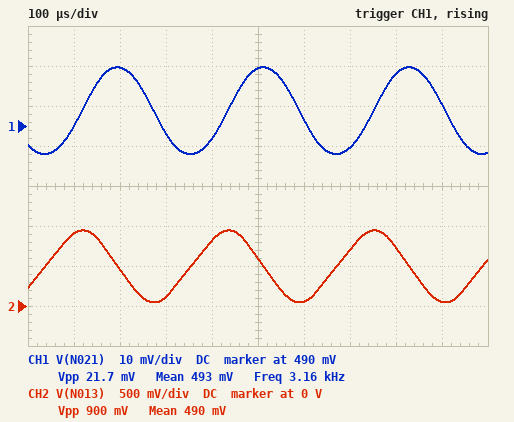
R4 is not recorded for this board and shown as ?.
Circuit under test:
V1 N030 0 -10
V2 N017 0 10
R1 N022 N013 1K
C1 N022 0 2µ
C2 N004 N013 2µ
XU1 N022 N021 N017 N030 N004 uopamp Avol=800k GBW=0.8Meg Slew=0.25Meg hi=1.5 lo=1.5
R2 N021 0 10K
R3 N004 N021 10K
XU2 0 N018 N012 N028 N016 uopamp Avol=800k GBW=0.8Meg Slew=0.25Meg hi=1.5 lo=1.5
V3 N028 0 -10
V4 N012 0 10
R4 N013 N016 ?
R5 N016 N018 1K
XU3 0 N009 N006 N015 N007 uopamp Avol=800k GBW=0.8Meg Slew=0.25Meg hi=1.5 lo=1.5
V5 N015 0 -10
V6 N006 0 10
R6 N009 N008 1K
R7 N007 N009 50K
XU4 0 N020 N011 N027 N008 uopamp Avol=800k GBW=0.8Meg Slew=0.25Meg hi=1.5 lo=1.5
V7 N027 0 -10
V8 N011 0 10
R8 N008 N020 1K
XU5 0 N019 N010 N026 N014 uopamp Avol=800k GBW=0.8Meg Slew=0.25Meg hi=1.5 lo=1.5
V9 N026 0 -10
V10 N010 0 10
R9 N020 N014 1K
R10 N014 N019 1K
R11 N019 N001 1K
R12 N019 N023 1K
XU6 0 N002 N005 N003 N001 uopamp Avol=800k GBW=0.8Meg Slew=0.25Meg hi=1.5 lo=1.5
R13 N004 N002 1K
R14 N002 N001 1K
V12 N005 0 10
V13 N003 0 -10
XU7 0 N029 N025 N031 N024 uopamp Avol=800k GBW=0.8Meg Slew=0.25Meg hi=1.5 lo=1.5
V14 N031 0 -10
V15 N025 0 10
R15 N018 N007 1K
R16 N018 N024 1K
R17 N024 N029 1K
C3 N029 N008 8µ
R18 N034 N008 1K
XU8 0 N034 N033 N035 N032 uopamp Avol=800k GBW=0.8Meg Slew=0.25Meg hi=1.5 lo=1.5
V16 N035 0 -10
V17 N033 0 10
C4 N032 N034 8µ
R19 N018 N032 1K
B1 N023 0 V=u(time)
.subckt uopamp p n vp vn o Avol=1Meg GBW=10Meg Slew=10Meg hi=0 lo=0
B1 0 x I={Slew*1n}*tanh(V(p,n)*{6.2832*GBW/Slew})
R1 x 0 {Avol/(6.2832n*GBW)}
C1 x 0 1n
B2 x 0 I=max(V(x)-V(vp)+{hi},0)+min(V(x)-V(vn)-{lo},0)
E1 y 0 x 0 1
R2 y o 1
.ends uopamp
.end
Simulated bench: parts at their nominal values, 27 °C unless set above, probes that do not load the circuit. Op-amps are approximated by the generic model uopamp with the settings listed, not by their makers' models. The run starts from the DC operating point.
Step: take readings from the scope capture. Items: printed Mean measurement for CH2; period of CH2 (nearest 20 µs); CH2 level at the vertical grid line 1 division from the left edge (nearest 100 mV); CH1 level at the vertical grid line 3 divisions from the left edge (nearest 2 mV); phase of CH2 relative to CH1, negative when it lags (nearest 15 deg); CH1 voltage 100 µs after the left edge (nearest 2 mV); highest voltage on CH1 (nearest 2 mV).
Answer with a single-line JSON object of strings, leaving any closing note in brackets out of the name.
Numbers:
{"printed Mean measurement for CH2": "490 mV", "period of CH2": "320 µs", "CH2 level at the vertical grid line 1 division from the left edge": "900 mV", "CH1 level at the vertical grid line 3 divisions from the left edge": "488 mV", "phase of CH2 relative to CH1, negative when it lags": "90 deg", "CH1 voltage 100 µs after the left edge": "490 mV", "highest voltage on CH1": "504 mV"}
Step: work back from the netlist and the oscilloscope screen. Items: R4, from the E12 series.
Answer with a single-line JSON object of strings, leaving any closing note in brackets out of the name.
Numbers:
{"R4, from the E12 series": "560 Ω"}
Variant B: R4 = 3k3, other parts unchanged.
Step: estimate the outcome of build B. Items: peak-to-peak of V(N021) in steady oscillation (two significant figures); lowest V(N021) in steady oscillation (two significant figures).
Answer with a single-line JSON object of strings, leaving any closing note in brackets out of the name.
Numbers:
{"peak-to-peak of V(N021) in steady oscillation": "2.5 mV", "lowest V(N021) in steady oscillation": "500 mV"}
